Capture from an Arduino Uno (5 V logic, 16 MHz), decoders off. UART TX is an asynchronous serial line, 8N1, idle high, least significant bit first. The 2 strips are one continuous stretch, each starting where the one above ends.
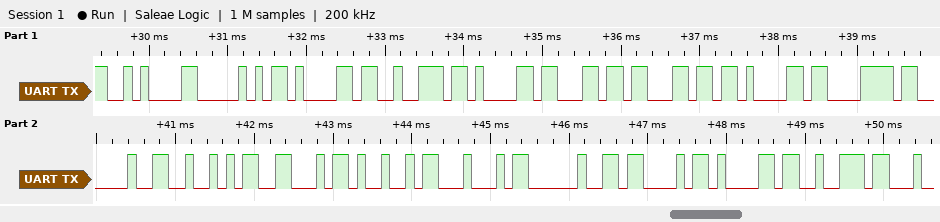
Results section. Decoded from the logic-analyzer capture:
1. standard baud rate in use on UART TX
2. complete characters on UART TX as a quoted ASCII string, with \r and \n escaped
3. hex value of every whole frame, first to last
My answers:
9600 baud
"\nParallax RFID Car"
0A 50 61 72 61 6C 6C 61 78 20 52 46 49 44 20 43 61 72
